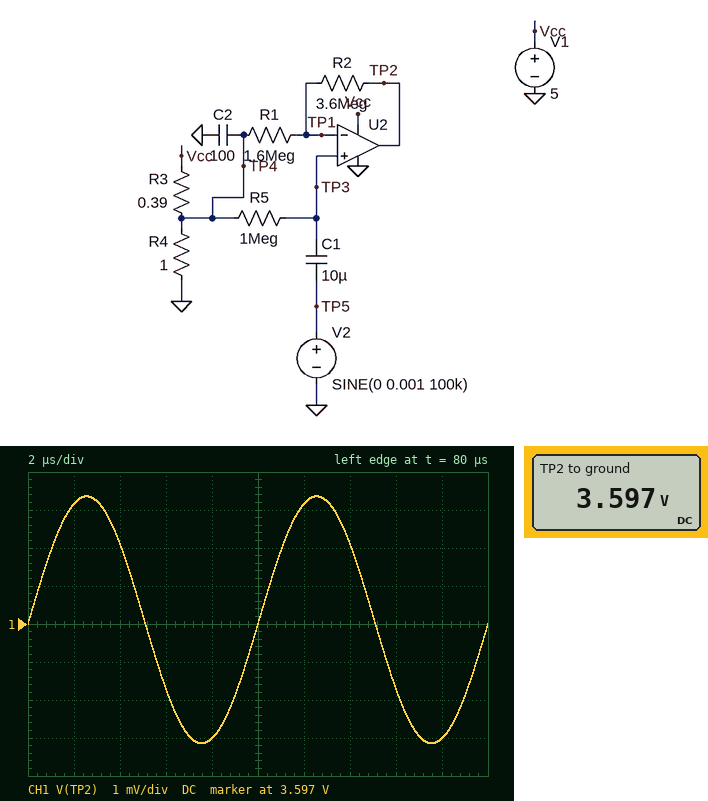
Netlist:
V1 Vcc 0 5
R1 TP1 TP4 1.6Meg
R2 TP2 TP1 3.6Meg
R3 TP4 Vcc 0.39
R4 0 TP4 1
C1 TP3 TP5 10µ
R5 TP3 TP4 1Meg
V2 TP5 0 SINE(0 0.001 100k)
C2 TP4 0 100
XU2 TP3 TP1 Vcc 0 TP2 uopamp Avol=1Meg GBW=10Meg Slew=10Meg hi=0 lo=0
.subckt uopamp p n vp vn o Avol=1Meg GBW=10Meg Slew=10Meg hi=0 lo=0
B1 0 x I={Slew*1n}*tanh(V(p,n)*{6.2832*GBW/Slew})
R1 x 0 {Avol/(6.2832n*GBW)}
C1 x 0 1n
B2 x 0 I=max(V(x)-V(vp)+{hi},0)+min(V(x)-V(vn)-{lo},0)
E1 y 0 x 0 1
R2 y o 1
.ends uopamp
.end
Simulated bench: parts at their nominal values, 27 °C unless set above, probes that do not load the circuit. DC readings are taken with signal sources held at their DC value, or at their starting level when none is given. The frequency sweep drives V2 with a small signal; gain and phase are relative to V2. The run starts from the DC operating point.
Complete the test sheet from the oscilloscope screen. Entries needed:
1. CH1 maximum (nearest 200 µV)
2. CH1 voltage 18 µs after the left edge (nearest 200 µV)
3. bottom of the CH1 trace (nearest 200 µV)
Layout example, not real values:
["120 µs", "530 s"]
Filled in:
["3.6004 V", "3.5940 V", "3.5938 V"]
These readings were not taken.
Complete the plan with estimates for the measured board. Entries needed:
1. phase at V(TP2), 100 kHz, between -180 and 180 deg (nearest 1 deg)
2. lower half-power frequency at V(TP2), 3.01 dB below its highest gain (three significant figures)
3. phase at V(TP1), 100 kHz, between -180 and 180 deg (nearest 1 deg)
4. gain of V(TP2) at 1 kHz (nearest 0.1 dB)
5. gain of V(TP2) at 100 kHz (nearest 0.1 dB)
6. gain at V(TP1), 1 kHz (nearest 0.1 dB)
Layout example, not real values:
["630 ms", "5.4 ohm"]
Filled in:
["-2 deg", "15.9 mHz", "-2 deg", "10.2 dB", "10.2 dB", "0 dB"]
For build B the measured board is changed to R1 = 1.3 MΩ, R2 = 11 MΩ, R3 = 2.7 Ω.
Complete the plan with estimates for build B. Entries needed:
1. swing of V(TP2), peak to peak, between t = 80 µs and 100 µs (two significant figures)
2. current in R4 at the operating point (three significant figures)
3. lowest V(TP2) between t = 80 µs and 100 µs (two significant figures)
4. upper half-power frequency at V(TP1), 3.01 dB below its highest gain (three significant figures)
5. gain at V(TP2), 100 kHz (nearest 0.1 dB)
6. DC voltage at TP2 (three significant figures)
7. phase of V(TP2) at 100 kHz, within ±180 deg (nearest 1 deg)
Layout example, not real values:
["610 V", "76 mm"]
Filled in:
["19 mV", "1.35 A", "1.3 V", "1.06 MHz", "19.5 dB", "1.35 V", "-5 deg"]
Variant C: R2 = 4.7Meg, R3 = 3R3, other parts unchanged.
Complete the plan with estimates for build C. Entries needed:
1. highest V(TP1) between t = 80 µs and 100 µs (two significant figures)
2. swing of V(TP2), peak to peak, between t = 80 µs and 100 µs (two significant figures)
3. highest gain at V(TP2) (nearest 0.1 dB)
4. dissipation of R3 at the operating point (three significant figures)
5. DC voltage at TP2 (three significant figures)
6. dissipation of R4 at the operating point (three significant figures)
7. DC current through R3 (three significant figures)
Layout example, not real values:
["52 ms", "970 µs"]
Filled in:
["1.2 V", "7.9 mV", "11.9 dB", "4.46 W", "1.16 V", "1.35 W", "1.16 A"]
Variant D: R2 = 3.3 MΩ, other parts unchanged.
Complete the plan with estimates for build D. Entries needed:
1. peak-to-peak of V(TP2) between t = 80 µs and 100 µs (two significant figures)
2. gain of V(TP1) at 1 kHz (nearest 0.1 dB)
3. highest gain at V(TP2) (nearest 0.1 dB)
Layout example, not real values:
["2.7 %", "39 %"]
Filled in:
["6.1 mV", "0 dB", "9.7 dB"]
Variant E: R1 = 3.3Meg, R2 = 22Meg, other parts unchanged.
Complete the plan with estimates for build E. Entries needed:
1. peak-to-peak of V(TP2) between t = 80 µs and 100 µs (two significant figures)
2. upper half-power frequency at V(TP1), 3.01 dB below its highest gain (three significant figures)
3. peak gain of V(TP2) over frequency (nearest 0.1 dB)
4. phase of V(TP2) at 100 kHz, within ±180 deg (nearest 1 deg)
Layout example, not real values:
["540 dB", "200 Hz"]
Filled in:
["15 mV", "1.30 MHz", "17.7 dB", "-4 deg"]
